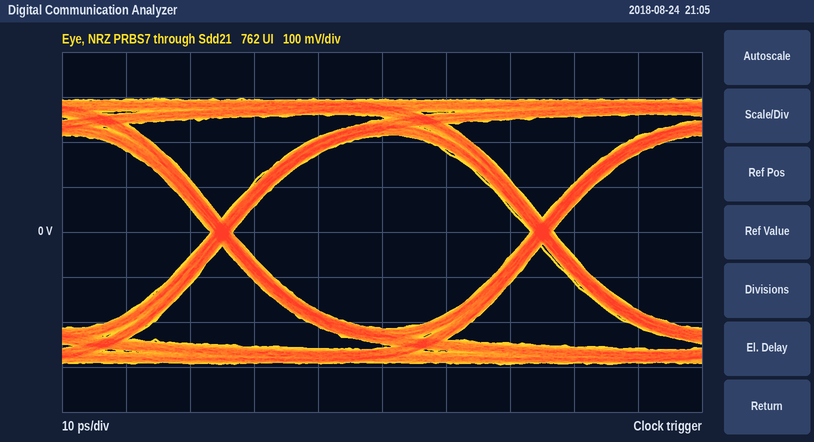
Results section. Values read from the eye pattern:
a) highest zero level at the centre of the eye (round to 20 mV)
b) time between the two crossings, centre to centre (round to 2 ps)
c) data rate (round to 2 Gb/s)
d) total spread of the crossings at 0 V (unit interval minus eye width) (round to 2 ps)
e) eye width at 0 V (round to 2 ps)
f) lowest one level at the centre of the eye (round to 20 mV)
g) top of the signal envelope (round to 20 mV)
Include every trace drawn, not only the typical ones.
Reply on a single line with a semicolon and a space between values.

-220 mV; 50 ps; 20 Gb/s; 4 ps; 46 ps; 220 mV; 300 mV
